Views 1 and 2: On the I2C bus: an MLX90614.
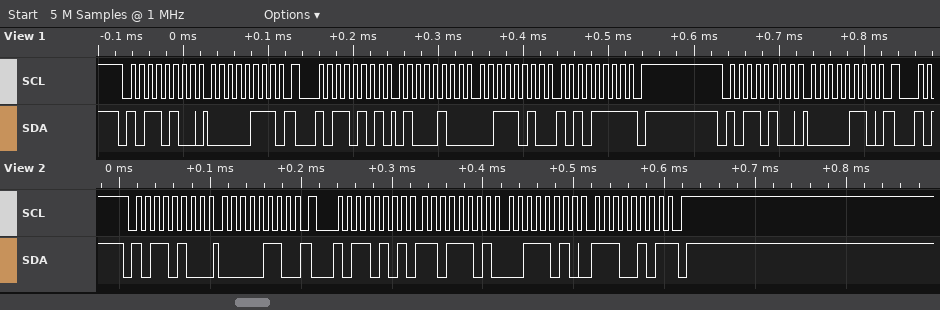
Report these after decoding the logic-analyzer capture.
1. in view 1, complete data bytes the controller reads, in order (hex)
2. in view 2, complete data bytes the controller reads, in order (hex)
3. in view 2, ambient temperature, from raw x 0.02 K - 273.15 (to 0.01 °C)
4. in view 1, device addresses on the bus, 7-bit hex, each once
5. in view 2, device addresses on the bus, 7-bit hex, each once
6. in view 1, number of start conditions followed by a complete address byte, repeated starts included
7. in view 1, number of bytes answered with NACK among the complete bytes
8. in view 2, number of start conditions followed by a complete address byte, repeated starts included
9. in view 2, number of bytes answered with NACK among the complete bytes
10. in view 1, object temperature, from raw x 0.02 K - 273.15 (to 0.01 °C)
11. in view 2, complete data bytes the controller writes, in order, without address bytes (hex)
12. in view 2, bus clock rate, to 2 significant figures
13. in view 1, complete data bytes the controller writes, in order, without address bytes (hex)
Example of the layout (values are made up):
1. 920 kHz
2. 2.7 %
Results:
1. 44 3A AF
2. DD 3A E5
3. 28.23 °C
4. 0x5A
5. 0x5A
6. 3
7. 1
8. 2
9. 1
10. 25.17 °C
11. 06
12. 100 kHz
13. 07 06
